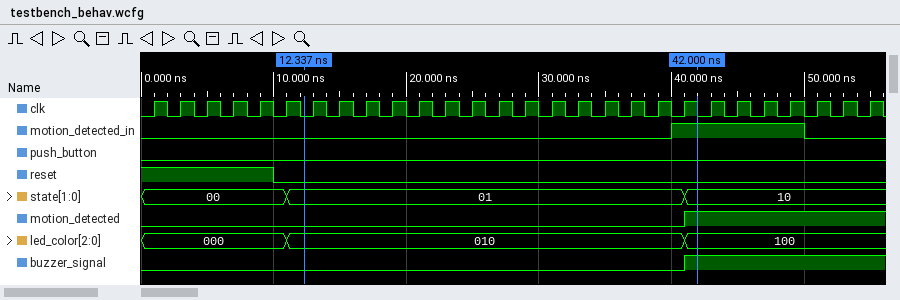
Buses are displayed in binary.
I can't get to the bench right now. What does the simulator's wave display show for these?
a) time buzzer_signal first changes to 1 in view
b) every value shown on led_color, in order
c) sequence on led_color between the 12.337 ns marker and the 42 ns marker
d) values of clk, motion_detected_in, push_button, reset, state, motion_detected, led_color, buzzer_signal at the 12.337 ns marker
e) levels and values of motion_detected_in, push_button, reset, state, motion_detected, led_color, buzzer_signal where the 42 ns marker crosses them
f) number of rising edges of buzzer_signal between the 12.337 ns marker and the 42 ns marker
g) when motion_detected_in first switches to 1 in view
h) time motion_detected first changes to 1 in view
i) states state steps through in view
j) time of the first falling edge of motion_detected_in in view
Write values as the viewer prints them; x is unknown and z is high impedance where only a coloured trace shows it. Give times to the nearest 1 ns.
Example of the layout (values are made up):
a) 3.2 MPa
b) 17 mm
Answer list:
a) 41 ns
b) 000, 010, 100
c) 010, 100
d) clk=0, motion_detected_in=0, push_button=0, reset=0, state=01, motion_detected=0, led_color=010, buzzer_signal=0
e) motion_detected_in=1, push_button=0, reset=0, state=10, motion_detected=1, led_color=100, buzzer_signal=1
f) 1
g) 40 ns
h) 41 ns
i) 00, 01, 10
j) 50 ns
